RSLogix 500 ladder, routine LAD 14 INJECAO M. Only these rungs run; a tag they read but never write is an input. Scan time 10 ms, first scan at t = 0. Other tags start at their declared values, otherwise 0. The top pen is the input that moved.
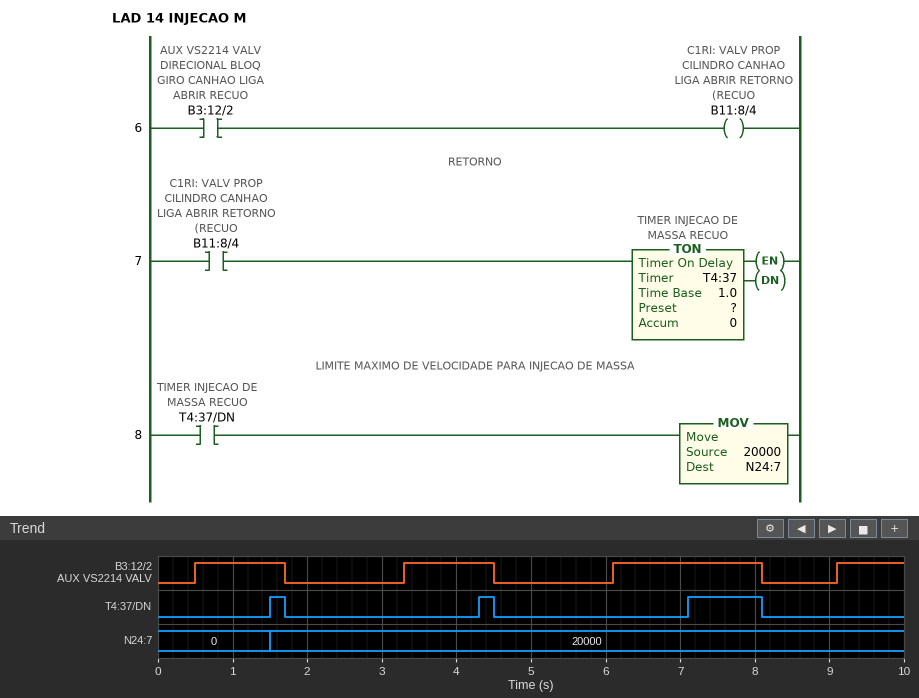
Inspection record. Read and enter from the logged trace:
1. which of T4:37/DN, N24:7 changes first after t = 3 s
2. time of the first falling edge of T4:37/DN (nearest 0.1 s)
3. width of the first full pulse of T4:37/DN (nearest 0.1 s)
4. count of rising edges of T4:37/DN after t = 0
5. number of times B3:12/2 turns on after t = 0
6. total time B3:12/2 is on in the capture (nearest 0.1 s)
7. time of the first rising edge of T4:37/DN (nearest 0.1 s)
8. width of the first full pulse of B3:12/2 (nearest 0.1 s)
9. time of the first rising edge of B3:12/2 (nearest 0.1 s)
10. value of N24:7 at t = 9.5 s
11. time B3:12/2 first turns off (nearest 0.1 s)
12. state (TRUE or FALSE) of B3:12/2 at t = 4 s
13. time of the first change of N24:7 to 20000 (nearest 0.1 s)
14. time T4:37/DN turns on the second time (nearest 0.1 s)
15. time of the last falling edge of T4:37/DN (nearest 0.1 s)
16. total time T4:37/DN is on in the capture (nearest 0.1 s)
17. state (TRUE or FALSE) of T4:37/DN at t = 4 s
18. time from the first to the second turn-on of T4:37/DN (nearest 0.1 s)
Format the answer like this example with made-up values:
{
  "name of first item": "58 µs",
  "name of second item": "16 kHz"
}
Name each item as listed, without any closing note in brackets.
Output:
{
  "which of T4:37/DN, N24:7 changes first after t = 3 s": "T4:37/DN",
  "time of the first falling edge of T4:37/DN": "1.7 s",
  "width of the first full pulse of T4:37/DN": "0.2 s",
  "count of rising edges of T4:37/DN after t = 0": "3",
  "number of times B3:12/2 turns on after t = 0": "4",
  "total time B3:12/2 is on in the capture": "5.3 s",
  "time of the first rising edge of T4:37/DN": "1.5 s",
  "width of the first full pulse of B3:12/2": "1.2 s",
  "time of the first rising edge of B3:12/2": "0.5 s",
  "value of N24:7 at t = 9.5 s": "20000",
  "time B3:12/2 first turns off": "1.7 s",
  "state (TRUE or FALSE) of B3:12/2 at t = 4 s": "TRUE",
  "time of the first change of N24:7 to 20000": "1.5 s",
  "time T4:37/DN turns on the second time": "4.3 s",
  "time of the last falling edge of T4:37/DN": "8.1 s",
  "total time T4:37/DN is on in the capture": "1.4 s",
  "state (TRUE or FALSE) of T4:37/DN at t = 4 s": "FALSE",
  "time from the first to the second turn-on of T4:37/DN": "2.8 s"
}
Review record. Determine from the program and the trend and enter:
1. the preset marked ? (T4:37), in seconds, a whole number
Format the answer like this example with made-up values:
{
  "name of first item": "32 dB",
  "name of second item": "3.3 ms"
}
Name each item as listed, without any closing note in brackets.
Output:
{
  "the preset marked ? (T4:37), in seconds, a whole number": "1 s"
}
